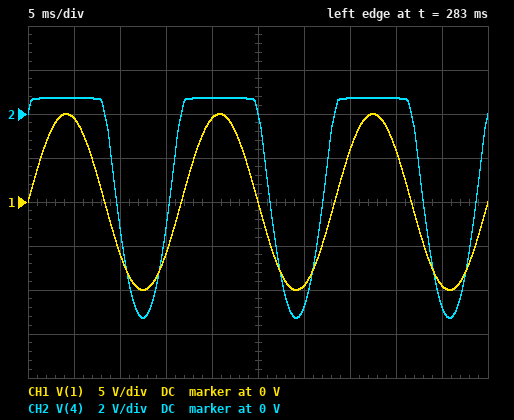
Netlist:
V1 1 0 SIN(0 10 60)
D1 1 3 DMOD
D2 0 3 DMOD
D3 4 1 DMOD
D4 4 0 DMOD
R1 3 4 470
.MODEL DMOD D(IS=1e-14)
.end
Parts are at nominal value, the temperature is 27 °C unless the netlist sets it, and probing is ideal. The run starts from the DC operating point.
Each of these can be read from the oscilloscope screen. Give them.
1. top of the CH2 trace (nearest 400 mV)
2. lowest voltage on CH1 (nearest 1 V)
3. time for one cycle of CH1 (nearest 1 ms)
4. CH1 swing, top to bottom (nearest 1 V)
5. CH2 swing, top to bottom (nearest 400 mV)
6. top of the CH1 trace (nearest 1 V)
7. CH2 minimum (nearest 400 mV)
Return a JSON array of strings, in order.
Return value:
["800 mV", "-10 V", "17 ms", "20 V", "10.0 V", "10 V", "-9.2 V"]
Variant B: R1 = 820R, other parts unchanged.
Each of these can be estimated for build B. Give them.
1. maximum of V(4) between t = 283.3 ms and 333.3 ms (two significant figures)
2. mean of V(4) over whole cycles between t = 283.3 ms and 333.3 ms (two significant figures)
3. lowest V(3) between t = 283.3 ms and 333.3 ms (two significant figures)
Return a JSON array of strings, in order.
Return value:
["720 mV", "-2.5 V", "-720 mV"]
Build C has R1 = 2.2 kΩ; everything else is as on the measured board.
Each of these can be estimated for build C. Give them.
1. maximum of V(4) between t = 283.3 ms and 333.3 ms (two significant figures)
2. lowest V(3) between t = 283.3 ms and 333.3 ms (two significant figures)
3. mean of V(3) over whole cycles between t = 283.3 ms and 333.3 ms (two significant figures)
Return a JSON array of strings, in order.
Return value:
["690 mV", "-690 mV", "2.5 V"]
